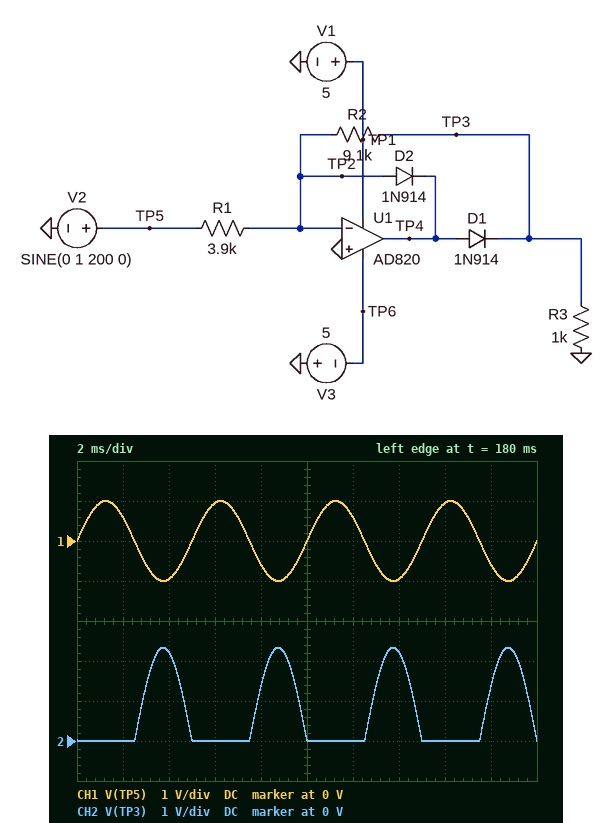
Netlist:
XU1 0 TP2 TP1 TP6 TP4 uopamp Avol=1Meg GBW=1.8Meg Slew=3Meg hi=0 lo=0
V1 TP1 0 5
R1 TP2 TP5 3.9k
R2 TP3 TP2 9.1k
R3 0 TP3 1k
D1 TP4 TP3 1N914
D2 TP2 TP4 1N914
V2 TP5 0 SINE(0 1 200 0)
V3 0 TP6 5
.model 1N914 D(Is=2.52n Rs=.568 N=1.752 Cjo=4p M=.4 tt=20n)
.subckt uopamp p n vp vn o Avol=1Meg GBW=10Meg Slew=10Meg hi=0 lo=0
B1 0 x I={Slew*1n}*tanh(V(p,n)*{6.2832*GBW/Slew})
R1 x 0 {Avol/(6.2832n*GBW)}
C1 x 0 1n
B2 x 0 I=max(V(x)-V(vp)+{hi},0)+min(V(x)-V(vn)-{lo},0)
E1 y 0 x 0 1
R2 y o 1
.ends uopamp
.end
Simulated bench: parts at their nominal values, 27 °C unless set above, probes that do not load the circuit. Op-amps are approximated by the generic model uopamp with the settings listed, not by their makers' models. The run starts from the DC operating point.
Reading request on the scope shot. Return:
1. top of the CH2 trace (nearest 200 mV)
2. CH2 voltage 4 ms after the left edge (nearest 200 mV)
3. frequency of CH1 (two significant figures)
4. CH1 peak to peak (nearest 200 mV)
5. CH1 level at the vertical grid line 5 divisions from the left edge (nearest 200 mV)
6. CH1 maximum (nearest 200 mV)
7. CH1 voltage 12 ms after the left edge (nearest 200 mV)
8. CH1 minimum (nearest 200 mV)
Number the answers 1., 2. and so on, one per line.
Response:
1. 2.4 V
2. 2.2 V
3. 200 Hz
4. 2.0 V
5. 0 V
6. 1.0 V
7. 600 mV
8. -1.0 V
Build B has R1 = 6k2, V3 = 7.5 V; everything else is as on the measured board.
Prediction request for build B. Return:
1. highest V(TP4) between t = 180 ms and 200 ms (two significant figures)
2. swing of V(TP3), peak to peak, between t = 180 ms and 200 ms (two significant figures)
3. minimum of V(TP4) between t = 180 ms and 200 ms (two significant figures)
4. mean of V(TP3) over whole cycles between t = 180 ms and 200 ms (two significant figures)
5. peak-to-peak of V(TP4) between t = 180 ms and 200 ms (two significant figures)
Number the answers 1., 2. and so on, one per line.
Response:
1. 2.1 V
2. 1.5 V
3. -500 mV
4. 470 mV
5. 2.6 V
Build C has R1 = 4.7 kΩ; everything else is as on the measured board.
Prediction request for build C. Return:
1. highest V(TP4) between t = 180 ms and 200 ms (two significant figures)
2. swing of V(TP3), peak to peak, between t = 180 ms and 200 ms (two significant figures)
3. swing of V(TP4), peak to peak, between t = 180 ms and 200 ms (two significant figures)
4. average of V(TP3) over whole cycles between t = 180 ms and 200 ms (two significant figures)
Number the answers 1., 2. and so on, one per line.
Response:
1. 2.6 V
2. 1.9 V
3. 3.1 V
4. 620 mV
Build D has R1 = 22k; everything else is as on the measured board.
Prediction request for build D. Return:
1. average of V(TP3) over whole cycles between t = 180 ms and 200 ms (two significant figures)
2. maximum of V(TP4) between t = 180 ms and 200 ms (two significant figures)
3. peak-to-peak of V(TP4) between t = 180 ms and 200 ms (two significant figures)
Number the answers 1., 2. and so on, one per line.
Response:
1. 130 mV
2. 960 mV
3. 1.4 V
